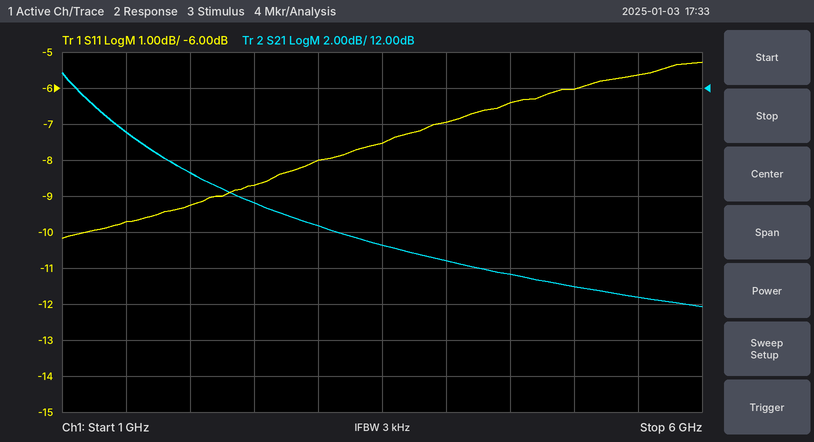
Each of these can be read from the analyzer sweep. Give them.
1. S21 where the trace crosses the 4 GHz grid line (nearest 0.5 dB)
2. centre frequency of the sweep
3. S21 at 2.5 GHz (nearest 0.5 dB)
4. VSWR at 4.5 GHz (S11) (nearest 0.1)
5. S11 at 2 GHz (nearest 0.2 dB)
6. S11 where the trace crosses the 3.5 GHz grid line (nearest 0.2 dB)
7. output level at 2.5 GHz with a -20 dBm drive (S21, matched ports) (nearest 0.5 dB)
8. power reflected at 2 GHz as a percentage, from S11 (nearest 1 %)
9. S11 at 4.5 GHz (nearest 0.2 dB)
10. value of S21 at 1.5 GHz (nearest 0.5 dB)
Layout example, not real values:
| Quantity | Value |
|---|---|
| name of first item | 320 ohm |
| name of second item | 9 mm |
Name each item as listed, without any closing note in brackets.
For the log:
| Quantity | Value |
|---|---|
| S21 where the trace crosses the 4 GHz grid line | 2.5 dB |
| centre frequency of the sweep | 3.5 GHz |
| S21 at 2.5 GHz | 5.5 dB |
| VSWR at 4.5 GHz (S11) | 2.8 |
| S11 at 2 GHz | -9.2 dB |
| S11 where the trace crosses the 3.5 GHz grid line | -7.6 dB |
| output level at 2.5 GHz with a -20 dBm drive (S21, matched ports) | -14.5 dBm |
| power reflected at 2 GHz as a percentage, from S11 | 12 % |
| S11 at 4.5 GHz | -6.4 dB |
| value of S21 at 1.5 GHz | 9.5 dB |
